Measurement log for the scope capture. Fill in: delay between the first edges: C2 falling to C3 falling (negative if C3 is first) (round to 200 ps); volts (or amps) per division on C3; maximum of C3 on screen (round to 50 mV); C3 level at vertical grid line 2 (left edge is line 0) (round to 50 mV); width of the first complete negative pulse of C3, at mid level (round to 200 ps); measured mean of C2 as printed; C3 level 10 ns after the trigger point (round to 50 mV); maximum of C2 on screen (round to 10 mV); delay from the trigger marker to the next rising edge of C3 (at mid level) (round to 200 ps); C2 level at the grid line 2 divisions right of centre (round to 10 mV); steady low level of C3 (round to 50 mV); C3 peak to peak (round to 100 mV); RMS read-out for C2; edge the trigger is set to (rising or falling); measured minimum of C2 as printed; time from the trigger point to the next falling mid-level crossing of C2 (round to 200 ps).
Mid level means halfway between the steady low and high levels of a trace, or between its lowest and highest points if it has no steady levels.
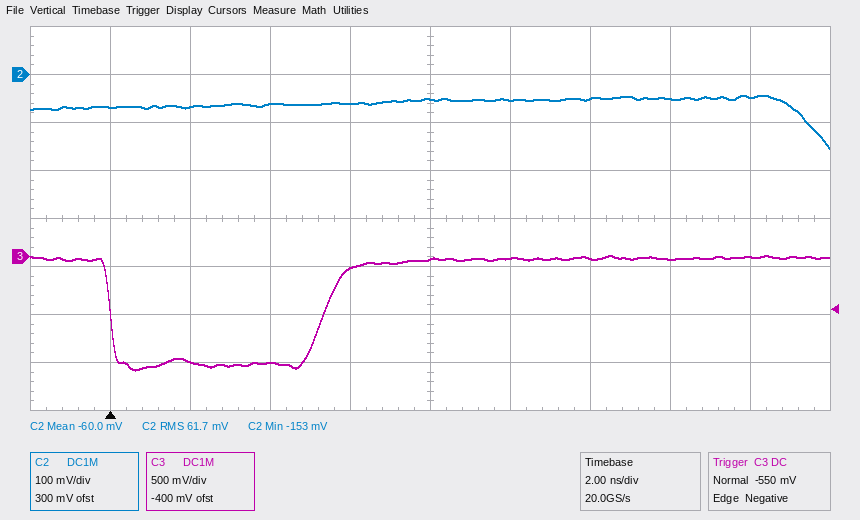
-17.4 ns
500 mV
0 mV
-1.10 V
5.4 ns
-60.0 mV
0 mV
-40 mV
5.4 ns
-50 mV
-1.10 V
1.20 V
61.7 mV
falling
-153 mV
17.4 ns
